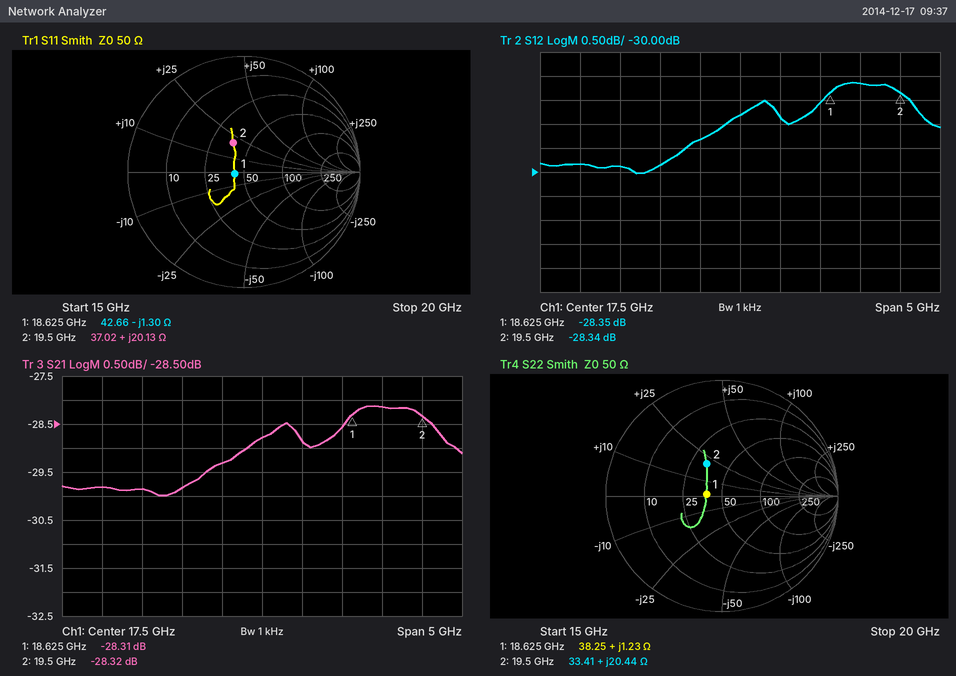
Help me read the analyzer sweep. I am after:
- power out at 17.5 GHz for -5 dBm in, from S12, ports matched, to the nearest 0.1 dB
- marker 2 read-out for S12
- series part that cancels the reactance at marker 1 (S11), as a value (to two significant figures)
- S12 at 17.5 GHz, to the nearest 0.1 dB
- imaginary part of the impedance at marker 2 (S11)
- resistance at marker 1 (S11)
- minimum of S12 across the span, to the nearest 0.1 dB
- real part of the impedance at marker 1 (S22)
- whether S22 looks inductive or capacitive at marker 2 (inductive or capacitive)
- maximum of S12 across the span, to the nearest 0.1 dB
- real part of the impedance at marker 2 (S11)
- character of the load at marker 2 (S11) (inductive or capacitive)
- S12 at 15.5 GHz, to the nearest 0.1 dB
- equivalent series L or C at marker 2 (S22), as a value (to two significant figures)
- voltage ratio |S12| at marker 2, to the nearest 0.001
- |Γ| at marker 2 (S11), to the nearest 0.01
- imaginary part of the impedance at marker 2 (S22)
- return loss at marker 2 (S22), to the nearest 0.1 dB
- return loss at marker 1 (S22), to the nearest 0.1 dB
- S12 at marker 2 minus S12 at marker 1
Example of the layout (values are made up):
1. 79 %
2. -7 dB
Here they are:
1. -33.8 dBm
2. -28.34 dB
3. 11 pH
4. -28.8 dB
5. +20.13 Ω
6. 42.66 Ω
7. -30.0 dB
8. 38.25 Ω
9. inductive
10. -28.1 dB
11. 37.02 Ω
12. inductive
13. -29.8 dB
14. 170 pH
15. 0.038
16. 0.27
17. +20.44 Ω
18. 10.3 dB
19. 17.5 dB
20. 0.01 dB
